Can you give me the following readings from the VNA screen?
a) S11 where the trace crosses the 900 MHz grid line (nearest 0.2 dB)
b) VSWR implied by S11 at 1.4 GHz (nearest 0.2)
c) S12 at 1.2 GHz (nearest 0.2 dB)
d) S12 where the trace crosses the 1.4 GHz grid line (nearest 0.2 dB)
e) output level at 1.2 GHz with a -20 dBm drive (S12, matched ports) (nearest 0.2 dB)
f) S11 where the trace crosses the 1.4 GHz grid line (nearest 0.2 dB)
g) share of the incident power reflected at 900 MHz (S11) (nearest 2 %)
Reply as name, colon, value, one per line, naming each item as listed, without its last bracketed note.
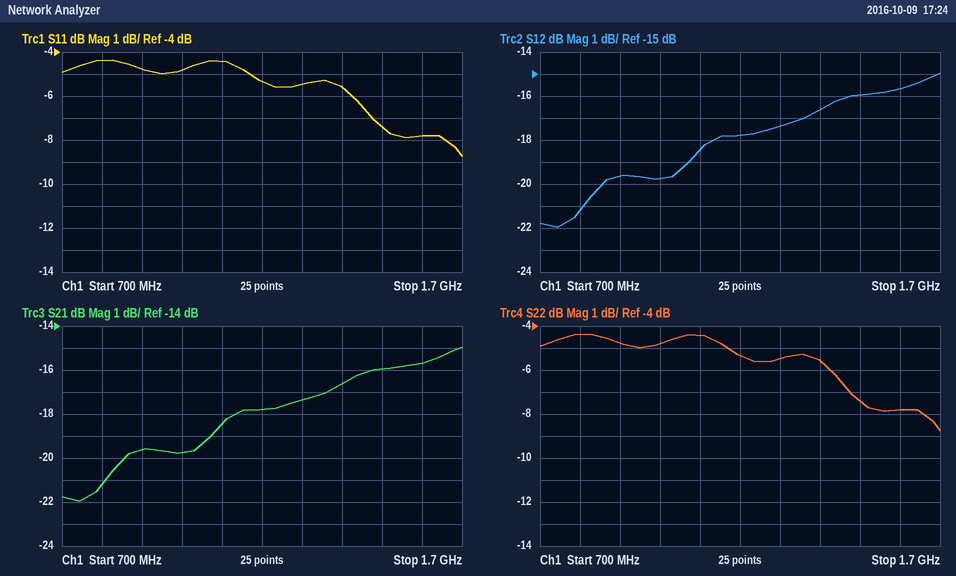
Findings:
S11 where the trace crosses the 900 MHz grid line: -4.8 dB
VSWR implied by S11 at 1.4 GHz: 3.2
S12 at 1.2 GHz: -17.8 dB
S12 where the trace crosses the 1.4 GHz grid line: -16.6 dB
output level at 1.2 GHz with a -20 dBm drive (S12, matched ports): -37.8 dBm
S11 where the trace crosses the 1.4 GHz grid line: -5.6 dB
share of the incident power reflected at 900 MHz (S11): 34 %
